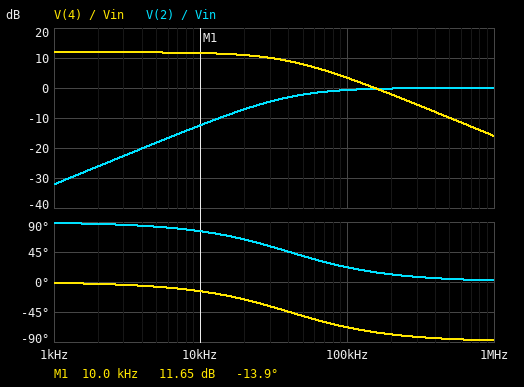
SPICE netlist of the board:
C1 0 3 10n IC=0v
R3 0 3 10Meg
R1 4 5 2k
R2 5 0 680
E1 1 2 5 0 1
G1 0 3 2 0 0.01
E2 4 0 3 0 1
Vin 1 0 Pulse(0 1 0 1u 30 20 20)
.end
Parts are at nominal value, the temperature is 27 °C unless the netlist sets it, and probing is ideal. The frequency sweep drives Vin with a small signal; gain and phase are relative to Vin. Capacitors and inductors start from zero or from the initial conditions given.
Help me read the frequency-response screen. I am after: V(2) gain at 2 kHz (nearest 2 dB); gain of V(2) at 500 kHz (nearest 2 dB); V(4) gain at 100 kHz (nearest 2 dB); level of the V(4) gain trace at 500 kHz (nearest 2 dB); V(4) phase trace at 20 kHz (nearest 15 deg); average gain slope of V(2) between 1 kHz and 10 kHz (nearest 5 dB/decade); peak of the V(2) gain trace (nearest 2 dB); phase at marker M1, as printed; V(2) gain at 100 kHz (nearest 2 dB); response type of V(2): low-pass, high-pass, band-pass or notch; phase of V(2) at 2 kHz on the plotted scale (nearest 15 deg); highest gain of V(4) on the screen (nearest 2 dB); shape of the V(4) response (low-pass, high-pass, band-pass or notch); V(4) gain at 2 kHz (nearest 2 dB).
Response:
-26 dB
0 dB
4 dB
-10 dB
-30 deg
20 dB/decade
0 dB
-13.9 deg
0 dB
high-pass
90 deg
12 dB
low-pass
12 dB
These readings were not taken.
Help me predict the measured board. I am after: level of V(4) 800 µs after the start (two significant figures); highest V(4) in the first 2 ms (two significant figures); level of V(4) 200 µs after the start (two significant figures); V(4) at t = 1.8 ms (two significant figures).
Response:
3.9 V
3.9 V
3.9 V
3.9 V
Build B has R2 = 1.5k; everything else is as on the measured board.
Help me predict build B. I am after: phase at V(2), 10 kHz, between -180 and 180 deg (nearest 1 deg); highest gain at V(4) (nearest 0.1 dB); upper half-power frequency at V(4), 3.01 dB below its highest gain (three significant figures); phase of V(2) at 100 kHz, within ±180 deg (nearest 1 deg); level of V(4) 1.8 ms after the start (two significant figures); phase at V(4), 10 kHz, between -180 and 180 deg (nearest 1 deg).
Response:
82 deg
7.4 dB
68.2 kHz
34 deg
2.3 V
-8 deg
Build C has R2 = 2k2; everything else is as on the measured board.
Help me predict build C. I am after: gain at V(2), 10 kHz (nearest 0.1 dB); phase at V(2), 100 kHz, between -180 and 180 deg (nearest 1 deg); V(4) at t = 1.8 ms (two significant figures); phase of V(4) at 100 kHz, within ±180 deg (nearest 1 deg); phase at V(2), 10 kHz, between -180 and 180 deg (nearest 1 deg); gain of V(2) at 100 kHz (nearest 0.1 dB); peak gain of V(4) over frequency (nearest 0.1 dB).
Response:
-18.5 dB
40 deg
1.9 V
-50 deg
83 deg
-2.3 dB
5.6 dB
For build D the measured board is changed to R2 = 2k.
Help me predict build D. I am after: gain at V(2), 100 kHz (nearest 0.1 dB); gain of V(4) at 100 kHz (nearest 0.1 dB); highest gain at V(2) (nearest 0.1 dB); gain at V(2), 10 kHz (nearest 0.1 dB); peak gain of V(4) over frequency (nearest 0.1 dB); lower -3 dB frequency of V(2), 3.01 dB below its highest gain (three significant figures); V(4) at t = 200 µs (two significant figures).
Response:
-2.1 dB
1.9 dB
0 dB
-18.1 dB
6.0 dB
79.6 kHz
2.0 V
